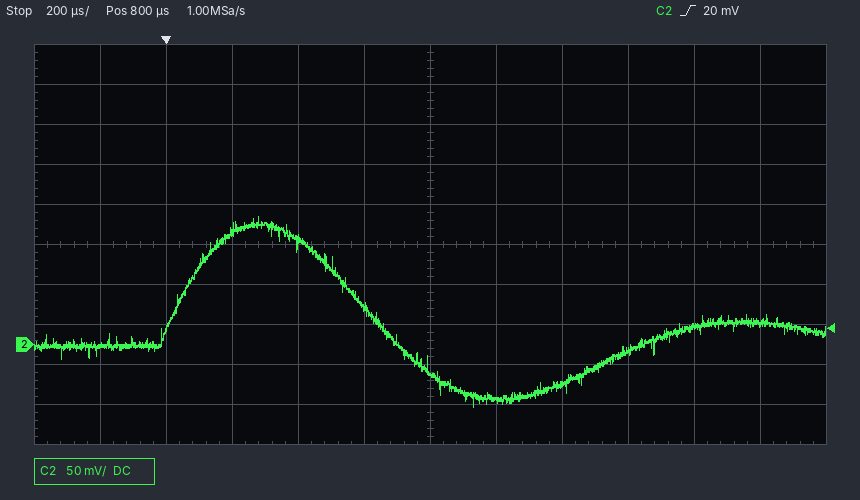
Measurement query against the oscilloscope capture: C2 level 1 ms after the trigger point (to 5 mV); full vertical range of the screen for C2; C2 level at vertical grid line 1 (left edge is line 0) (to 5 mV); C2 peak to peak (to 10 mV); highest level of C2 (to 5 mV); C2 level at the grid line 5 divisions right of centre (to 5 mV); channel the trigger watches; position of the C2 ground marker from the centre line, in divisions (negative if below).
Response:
-70 mV
500 mV
0 mV
240 mV
160 mV
25 mV
C2
-2.5 div
